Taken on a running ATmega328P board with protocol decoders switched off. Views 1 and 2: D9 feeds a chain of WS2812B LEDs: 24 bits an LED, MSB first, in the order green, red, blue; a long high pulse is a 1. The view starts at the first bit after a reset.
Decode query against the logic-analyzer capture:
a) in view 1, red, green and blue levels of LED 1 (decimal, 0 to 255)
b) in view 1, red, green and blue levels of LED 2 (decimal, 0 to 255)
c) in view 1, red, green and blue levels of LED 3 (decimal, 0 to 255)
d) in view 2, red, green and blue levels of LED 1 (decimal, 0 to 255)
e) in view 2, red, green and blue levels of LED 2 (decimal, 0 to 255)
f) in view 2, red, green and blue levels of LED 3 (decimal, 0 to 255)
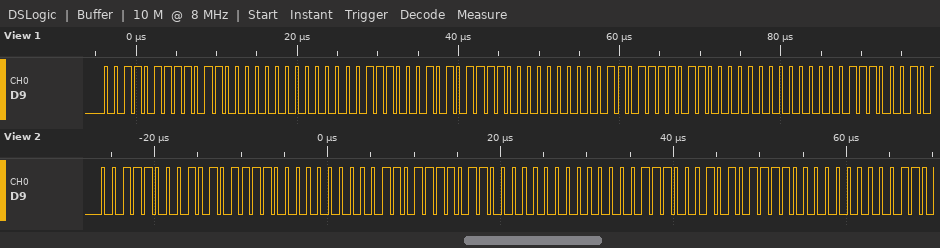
176, 55, 0
175, 56, 0
176, 55, 0
175, 56, 0
176, 55, 0
175, 56, 0
